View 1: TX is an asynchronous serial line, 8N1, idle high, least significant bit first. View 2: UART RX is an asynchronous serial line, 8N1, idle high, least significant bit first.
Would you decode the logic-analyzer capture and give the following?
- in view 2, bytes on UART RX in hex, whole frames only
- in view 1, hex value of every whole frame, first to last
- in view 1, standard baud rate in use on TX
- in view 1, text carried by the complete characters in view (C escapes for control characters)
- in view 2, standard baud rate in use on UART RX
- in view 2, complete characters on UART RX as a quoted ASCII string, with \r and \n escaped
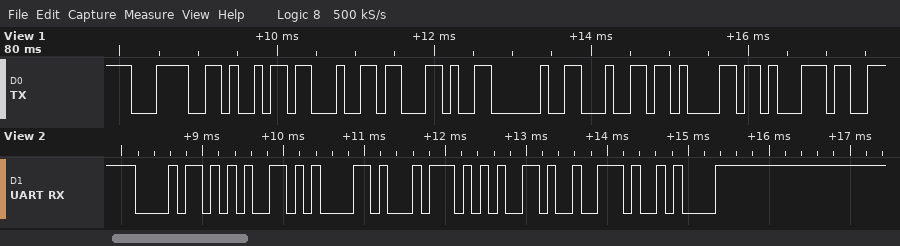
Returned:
68 65 61 74 65 72 0A
0x3C 0x69 0x64 0x2C 0x20 0x64 0x61 0x71
9600 baud
"<id, daq"
9600 baud
"heater\n"
